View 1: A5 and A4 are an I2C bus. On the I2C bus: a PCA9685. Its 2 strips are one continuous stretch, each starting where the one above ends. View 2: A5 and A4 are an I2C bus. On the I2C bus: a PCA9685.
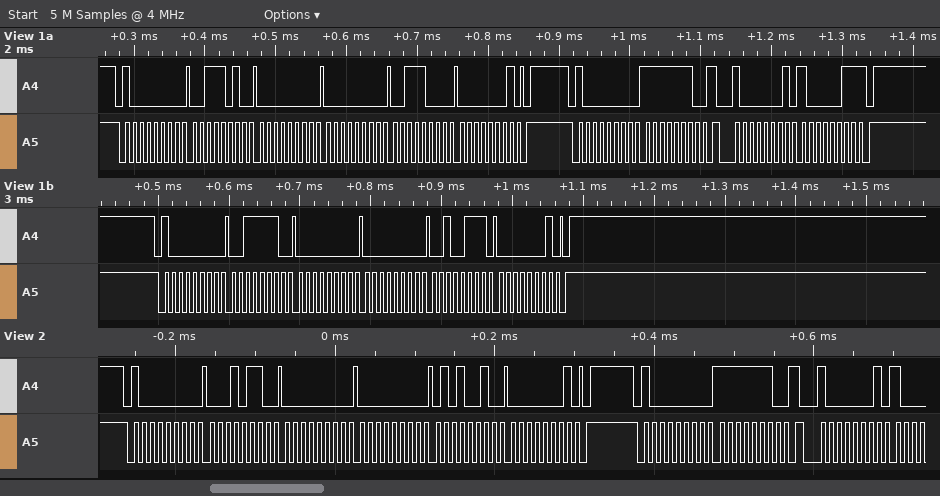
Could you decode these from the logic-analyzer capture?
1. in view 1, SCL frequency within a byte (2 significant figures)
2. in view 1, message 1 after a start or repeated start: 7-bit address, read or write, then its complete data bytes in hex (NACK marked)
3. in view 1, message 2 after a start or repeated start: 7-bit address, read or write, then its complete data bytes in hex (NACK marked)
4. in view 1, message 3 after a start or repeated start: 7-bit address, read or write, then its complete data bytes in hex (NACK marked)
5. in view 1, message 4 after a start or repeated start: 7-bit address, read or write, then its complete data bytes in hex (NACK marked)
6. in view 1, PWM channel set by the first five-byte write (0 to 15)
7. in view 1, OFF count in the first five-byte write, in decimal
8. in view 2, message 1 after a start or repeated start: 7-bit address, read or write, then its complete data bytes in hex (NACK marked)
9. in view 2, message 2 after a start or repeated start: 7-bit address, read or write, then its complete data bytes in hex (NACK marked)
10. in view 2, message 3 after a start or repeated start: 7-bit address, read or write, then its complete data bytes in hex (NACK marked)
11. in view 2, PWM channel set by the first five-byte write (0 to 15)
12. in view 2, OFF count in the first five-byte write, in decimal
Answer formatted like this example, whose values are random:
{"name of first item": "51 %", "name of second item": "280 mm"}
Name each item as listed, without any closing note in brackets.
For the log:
{"in view 1, SCL frequency within a byte": "100 kHz", "in view 1, message 1 after a start or repeated start: 7-bit address, read or write, then its complete data bytes in hex": "0x40 write: 3A 00 00 38 01", "in view 1, message 2 after a start or repeated start: 7-bit address, read or write, then its complete data bytes in hex": "0x40 write: FE", "in view 1, message 3 after a start or repeated start: 7-bit address, read or write, then its complete data bytes in hex": "0x40 read: 83 NACK", "in view 1, message 4 after a start or repeated start: 7-bit address, read or write, then its complete data bytes in hex": "0x40 write: 3E 00 00 27 01", "in view 1, PWM channel set by the first five-byte write": "13", "in view 1, OFF count in the first five-byte write, in decimal": "312", "in view 2, message 1 after a start or repeated start: 7-bit address, read or write, then its complete data bytes in hex": "0x40 write: 16 00 00 52 01", "in view 2, message 2 after a start or repeated start: 7-bit address, read or write, then its complete data bytes in hex": "0x40 write: FE", "in view 2, message 3 after a start or repeated start: 7-bit address, read or write, then its complete data bytes in hex": "0x40 read", "in view 2, PWM channel set by the first five-byte write": "4", "in view 2, OFF count in the first five-byte write, in decimal": "338"}
